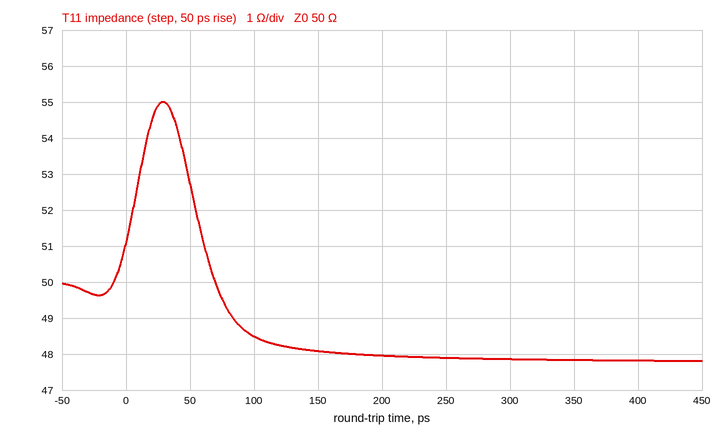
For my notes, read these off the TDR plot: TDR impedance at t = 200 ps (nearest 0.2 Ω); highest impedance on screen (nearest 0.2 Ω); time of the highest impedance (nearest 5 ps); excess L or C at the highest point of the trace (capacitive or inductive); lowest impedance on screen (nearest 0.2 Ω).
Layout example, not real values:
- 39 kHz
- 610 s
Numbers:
- 48.0 Ω
- 55.0 Ω
- 30 ps
- inductive
- 47.8 Ω
